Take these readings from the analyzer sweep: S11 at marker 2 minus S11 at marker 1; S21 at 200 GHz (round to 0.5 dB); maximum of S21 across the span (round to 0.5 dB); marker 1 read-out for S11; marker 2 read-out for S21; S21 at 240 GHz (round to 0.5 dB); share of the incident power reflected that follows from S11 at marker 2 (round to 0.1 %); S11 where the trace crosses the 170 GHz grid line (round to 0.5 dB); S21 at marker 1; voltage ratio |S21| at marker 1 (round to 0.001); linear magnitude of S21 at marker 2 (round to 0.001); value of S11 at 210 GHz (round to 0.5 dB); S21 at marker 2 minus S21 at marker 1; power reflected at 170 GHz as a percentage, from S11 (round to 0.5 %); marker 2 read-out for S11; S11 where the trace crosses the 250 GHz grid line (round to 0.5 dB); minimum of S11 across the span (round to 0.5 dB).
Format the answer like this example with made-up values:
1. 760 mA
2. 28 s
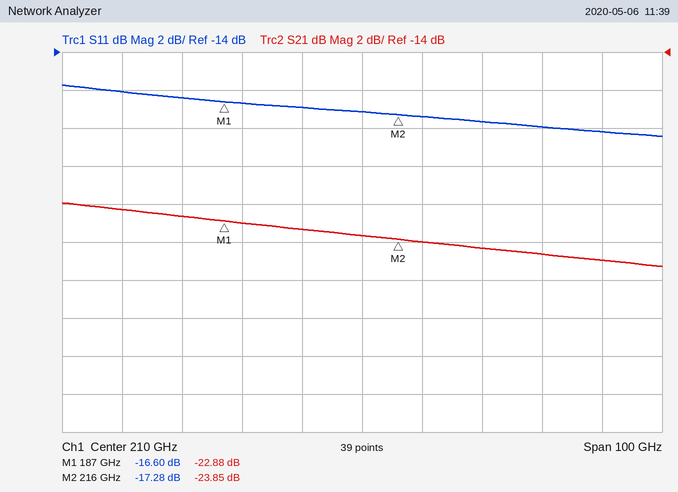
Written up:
1. -0.68 dB
2. -23.5 dB
3. -22.0 dB
4. -16.60 dB
5. -23.85 dB
6. -24.5 dB
7. 1.9 %
8. -16.0 dB
9. -22.88 dB
10. 0.072
11. 0.064
12. -17.0 dB
13. -0.97 dB
14. 2.5 %
15. -17.28 dB
16. -18.0 dB
17. -18.5 dB
